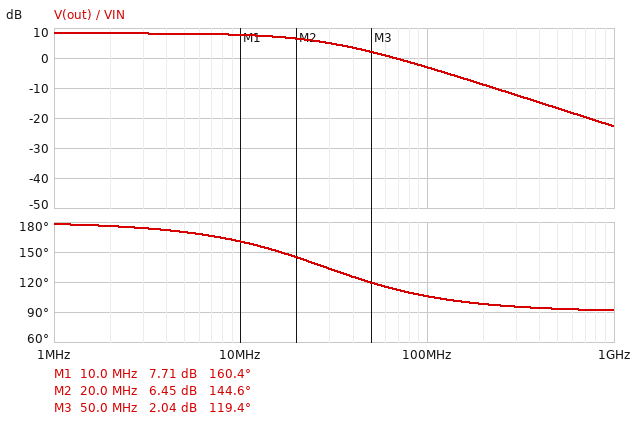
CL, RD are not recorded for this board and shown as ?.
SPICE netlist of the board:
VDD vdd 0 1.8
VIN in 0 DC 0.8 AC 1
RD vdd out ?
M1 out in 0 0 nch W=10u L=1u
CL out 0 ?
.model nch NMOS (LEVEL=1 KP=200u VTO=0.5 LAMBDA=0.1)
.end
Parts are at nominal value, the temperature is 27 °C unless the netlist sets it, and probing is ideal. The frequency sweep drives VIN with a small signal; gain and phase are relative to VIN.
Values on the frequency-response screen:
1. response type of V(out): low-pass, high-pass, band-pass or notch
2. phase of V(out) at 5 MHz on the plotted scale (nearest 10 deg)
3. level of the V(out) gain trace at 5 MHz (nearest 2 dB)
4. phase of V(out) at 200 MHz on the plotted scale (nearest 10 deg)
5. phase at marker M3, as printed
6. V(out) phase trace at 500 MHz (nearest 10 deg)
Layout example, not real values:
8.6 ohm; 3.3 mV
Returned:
low-pass; 170 deg; 8 dB; 100 deg; 119.4 deg; 90 deg
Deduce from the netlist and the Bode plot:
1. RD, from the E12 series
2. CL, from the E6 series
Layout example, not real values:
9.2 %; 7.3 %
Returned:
3.9 kΩ; 1.5 pF
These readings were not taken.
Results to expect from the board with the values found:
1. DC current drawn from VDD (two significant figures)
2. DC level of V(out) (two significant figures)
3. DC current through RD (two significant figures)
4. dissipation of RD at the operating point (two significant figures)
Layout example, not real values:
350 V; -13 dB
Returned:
100 µA; 1.4 V; 100 µA; 41 µW
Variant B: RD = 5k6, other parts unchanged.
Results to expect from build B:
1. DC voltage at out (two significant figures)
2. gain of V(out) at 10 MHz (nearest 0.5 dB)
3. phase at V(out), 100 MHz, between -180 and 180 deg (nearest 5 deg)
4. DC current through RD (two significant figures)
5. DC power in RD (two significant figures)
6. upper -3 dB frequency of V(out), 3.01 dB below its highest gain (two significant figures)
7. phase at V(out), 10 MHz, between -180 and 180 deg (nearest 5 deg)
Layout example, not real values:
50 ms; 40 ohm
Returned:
1.2 V; 10.0 dB; 100 deg; 100 µA; 57 µW; 20 MHz; 155 deg
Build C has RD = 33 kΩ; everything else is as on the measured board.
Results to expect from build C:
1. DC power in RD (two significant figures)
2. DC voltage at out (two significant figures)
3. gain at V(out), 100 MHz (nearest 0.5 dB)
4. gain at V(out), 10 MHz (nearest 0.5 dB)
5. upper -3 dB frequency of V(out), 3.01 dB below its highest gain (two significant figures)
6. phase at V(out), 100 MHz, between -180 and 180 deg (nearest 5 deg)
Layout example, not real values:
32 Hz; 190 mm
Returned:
87 µW; 100 mV; -14.0 dB; -6.5 dB; 46 MHz; 115 deg
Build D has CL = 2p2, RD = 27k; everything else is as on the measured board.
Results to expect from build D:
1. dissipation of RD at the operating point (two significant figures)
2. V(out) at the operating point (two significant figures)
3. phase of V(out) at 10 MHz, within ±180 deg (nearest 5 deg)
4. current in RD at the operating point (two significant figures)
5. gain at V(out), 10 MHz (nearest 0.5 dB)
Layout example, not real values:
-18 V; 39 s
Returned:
100 µW; 130 mV; 160 deg; 62 µA; -4.0 dB
